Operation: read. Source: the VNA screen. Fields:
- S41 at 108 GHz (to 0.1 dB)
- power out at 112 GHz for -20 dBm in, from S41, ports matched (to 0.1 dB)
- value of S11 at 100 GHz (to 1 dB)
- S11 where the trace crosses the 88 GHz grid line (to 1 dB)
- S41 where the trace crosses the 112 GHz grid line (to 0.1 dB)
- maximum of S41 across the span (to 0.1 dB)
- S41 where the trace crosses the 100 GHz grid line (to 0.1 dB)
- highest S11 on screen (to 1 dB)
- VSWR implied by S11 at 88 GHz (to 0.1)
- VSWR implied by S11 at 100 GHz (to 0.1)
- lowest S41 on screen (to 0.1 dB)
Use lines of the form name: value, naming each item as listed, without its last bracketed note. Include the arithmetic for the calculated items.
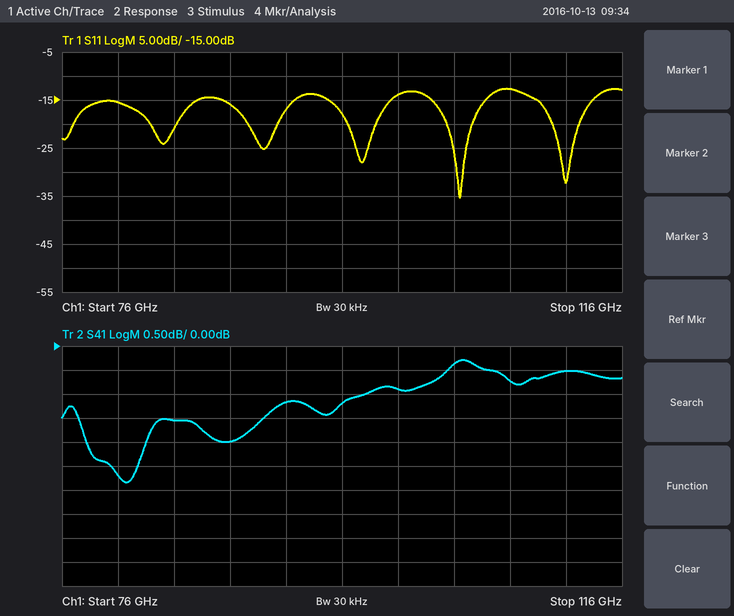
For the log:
S41 at 108 GHz: -0.7 dB
power out at 112 GHz for -20 dBm in, from S41, ports matched: -20 dBm + (-0.5 dB) = -20.5 dBm
value of S11 at 100 GHz: -14 dB
S11 where the trace crosses the 88 GHz grid line: -16 dB
S41 where the trace crosses the 112 GHz grid line: -0.5 dB
maximum of S41 across the span: -0.3 dB
S41 where the trace crosses the 100 GHz grid line: -0.9 dB
highest S11 on screen: -13 dB
VSWR implied by S11 at 88 GHz: |Γ| = 10^(-16/20) = 0.1585; VSWR = (1 + 0.1585)/(1 − 0.1585) ≈ 1.4
VSWR implied by S11 at 100 GHz: |Γ| = 10^(-14/20) = 0.1995; VSWR = (1 + 0.1995)/(1 − 0.1995) ≈ 1.5
lowest S41 on screen: -2.8 dB
